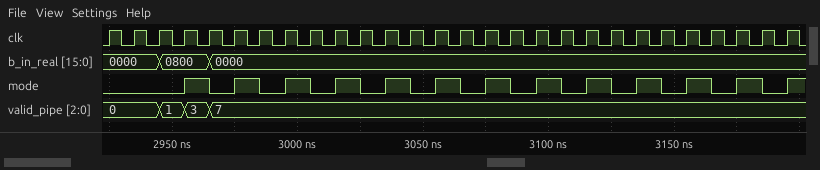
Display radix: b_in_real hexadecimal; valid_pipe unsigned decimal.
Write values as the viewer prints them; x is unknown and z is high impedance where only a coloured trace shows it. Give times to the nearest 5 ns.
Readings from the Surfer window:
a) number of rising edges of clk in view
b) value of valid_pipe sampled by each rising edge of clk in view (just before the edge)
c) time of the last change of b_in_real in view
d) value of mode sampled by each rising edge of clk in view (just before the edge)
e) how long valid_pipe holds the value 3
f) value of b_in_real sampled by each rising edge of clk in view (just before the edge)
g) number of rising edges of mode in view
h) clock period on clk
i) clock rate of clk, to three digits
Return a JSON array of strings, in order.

["28", "0, 0, 0, 1, 3, 7, 7, 7, 7, 7, 7, 7, 7, 7, 7, 7, 7, 7, 7, 7, 7, 7, 7, 7, 7, 7, 7, 7", "2965 ns", "0 0 0 0 1 0 1 0 1 0 1 0 1 0 1 0 1 0 1 0 1 0 1 0 1 0 1 0", "10 ns", "0000, 0000, 0000, 0800, 0800, 0000, 0000, 0000, 0000, 0000, 0000, 0000, 0000, 0000, 0000, 0000, 0000, 0000, 0000, 0000, 0000, 0000, 0000, 0000, 0000, 0000, 0000, 0000", "13", "10 ns", "100 MHz"]
